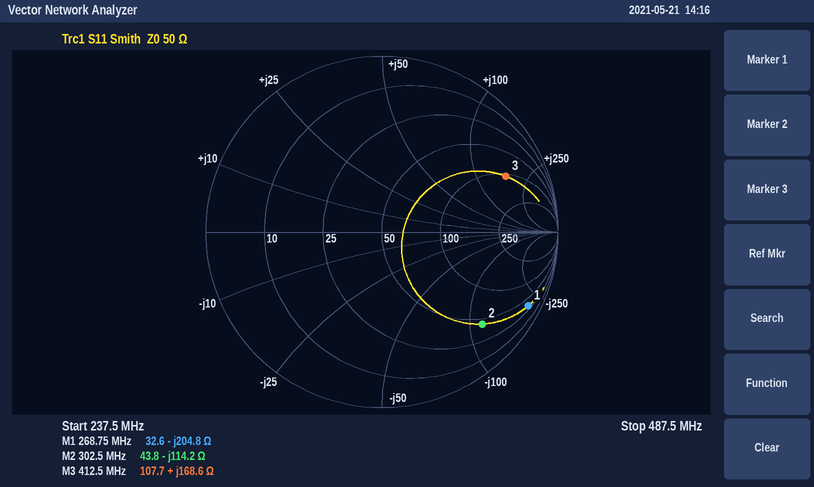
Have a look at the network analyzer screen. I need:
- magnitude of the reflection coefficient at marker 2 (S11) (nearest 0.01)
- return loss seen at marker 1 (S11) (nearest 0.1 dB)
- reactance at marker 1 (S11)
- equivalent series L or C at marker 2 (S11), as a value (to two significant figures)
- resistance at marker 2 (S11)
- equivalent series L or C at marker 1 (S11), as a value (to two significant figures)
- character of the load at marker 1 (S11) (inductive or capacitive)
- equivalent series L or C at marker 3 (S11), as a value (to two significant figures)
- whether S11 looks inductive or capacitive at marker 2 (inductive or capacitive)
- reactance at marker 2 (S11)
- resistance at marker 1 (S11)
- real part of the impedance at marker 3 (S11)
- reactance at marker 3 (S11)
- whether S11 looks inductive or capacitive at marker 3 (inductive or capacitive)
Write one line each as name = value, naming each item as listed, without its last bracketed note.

magnitude of the reflection coefficient at marker 2 (S11) = 0.77
return loss seen at marker 1 (S11) = 0.6 dB
reactance at marker 1 = -204.8 Ω
equivalent series L or C at marker 2 (S11), as a value = 4.6 pF
resistance at marker 2 = 43.8 Ω
equivalent series L or C at marker 1 (S11), as a value = 2.9 pF
character of the load at marker 1 (S11) = capacitive
equivalent series L or C at marker 3 (S11), as a value = 65 nH
whether S11 looks inductive or capacitive at marker 2 = capacitive
reactance at marker 2 = -114.2 Ω
resistance at marker 1 = 32.6 Ω
real part of the impedance at marker 3 = 107.7 Ω
reactance at marker 3 = +168.6 Ω
whether S11 looks inductive or capacitive at marker 3 = inductive
